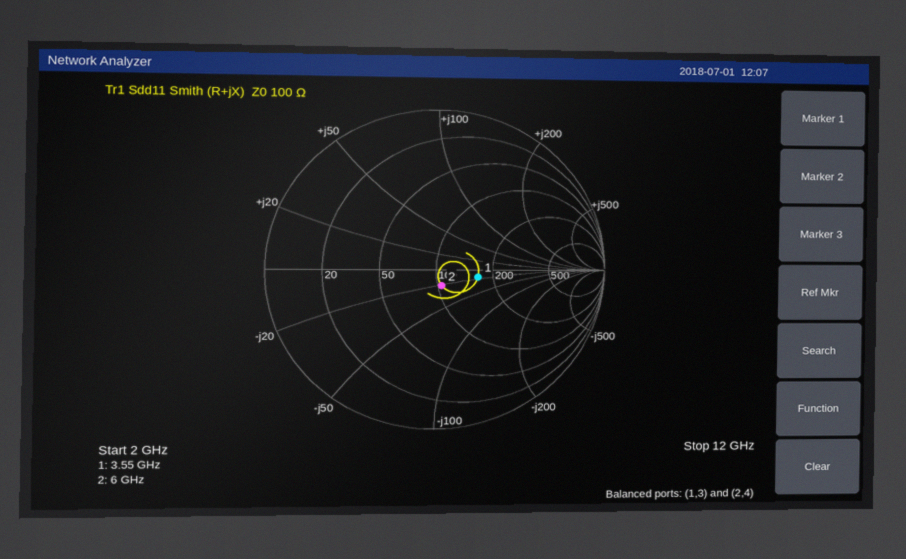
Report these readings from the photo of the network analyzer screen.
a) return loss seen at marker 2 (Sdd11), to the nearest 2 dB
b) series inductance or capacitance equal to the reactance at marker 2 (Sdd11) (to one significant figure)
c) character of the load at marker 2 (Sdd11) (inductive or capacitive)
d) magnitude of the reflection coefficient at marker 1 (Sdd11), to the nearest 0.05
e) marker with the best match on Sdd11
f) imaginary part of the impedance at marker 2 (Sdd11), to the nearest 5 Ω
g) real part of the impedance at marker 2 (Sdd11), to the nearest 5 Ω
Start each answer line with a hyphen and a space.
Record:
- 20 dB
- 1 pF
- capacitive
- 0.25
- marker 2
- -20 Ω
- 105 Ω
